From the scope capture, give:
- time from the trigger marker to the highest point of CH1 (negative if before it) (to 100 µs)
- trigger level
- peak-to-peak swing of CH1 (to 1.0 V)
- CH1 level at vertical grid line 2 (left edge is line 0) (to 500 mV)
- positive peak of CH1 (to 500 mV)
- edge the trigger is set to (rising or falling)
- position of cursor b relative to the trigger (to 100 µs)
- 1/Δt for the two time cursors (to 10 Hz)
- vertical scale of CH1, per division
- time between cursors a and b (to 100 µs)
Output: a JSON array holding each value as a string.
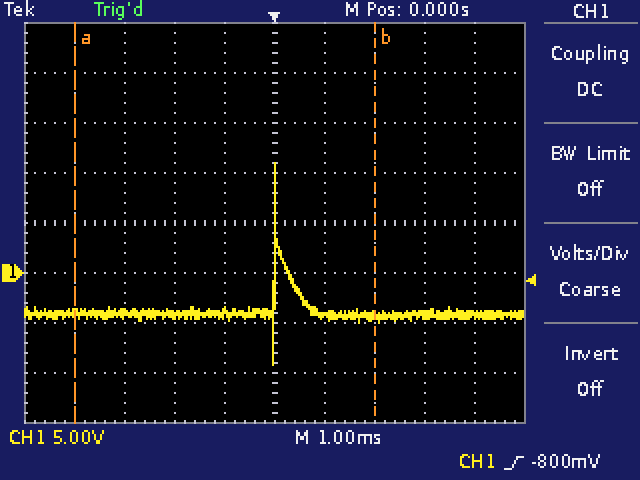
["0.0 ms", "-800 mV", "20.0 V", "-4.0 V", "11.0 V", "rising", "+2.0 ms", "170 Hz", "5 V", "6.0 ms"]
